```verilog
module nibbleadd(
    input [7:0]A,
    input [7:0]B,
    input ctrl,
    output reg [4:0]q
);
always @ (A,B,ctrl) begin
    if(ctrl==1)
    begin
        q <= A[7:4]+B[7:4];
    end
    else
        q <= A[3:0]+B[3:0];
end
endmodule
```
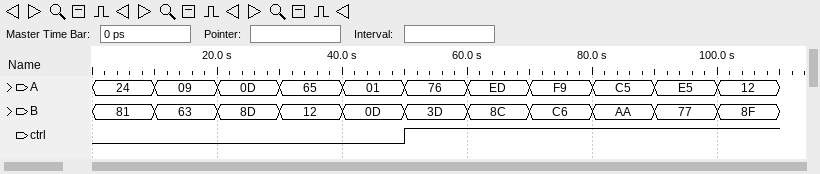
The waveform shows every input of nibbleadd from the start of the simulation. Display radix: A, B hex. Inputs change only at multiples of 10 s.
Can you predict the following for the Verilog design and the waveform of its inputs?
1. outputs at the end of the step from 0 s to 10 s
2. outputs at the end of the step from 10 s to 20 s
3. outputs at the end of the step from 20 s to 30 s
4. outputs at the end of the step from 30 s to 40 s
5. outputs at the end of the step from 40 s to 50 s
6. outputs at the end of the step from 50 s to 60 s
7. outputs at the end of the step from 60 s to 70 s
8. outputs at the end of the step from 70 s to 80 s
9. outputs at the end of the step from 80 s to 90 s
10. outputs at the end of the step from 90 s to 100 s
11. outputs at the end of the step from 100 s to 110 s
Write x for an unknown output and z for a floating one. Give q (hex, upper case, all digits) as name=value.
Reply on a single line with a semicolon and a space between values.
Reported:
q=05; q=0C; q=1A; q=07; q=0E; q=0A; q=16; q=1B; q=16; q=15; q=09
